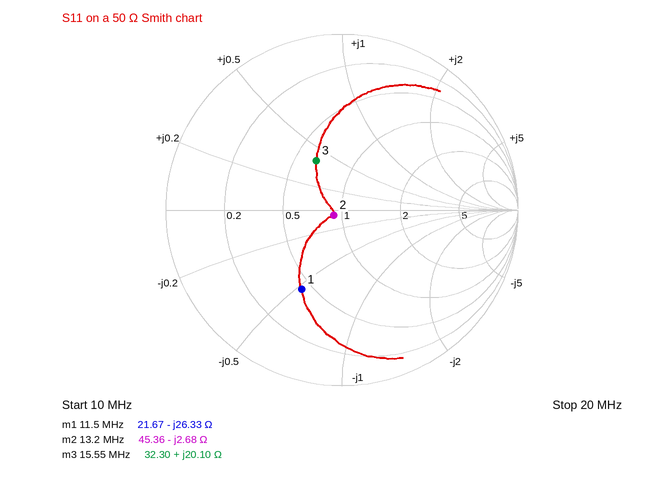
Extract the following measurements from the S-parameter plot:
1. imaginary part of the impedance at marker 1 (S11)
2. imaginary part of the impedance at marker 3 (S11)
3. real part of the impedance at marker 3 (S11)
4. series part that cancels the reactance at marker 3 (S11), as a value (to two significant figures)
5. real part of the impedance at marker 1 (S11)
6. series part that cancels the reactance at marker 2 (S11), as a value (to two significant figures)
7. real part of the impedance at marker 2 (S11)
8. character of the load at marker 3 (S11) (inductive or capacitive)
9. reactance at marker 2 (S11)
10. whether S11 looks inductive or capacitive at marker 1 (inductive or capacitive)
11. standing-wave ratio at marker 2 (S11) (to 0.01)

-26.33 Ω
+20.10 Ω
32.30 Ω
510 pF
21.67 Ω
32 nH
45.36 Ω
inductive
-2.68 Ω
capacitive
1.12
